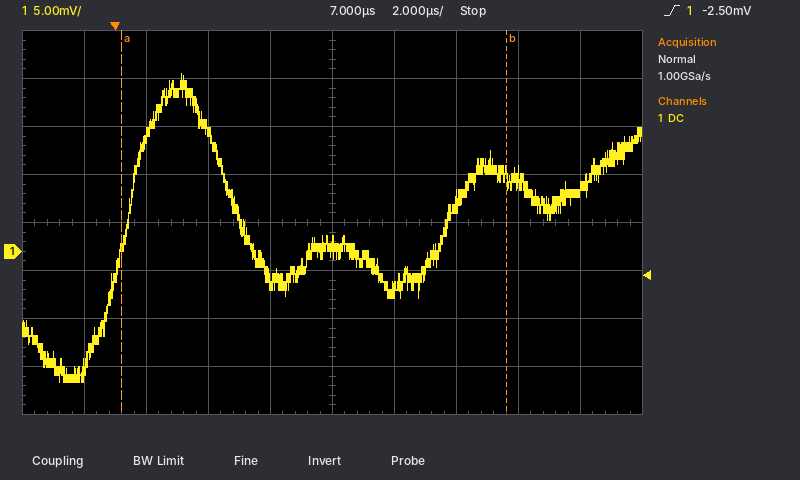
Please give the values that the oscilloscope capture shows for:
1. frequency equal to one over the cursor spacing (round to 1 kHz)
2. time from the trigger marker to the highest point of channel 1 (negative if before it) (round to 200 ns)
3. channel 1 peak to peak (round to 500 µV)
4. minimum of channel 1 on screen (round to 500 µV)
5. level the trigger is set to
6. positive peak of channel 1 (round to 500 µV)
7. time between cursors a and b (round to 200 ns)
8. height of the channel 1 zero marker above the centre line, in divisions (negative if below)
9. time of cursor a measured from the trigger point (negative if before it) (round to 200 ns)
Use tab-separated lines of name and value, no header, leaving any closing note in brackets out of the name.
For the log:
frequency equal to one over the cursor spacing	81 kHz
time from the trigger marker to the highest point of channel 1 (negative if before it)	+2.2 µs
channel 1 peak to peak	32.0 mV
minimum of channel 1 on screen	-13.5 mV
level the trigger is set to	-2.50 mV
positive peak of channel 1	18.5 mV
time between cursors a and b	12.4 µs
height of the channel 1 zero marker above the centre line, in divisions	-0.6 div
time of cursor a measured from the trigger point (negative if before it)	+200 ns
